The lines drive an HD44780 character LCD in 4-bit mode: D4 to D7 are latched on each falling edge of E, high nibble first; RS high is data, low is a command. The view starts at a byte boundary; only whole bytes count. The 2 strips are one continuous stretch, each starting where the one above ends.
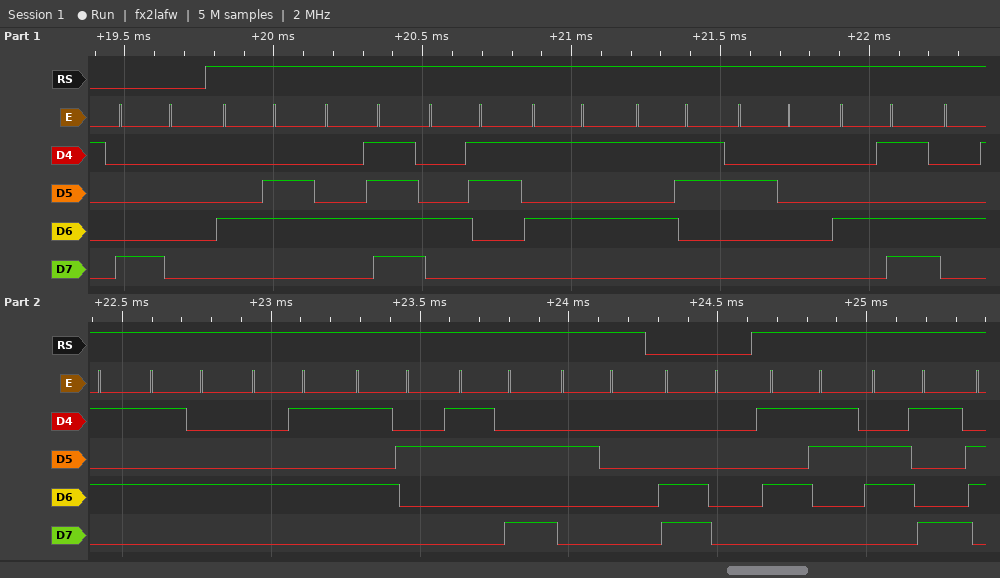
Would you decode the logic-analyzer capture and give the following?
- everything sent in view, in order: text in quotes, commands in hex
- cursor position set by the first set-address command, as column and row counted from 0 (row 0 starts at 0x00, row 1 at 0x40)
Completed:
0x80 "FOCUS METER: " 0xC0 "Si"
column 0, row 0
